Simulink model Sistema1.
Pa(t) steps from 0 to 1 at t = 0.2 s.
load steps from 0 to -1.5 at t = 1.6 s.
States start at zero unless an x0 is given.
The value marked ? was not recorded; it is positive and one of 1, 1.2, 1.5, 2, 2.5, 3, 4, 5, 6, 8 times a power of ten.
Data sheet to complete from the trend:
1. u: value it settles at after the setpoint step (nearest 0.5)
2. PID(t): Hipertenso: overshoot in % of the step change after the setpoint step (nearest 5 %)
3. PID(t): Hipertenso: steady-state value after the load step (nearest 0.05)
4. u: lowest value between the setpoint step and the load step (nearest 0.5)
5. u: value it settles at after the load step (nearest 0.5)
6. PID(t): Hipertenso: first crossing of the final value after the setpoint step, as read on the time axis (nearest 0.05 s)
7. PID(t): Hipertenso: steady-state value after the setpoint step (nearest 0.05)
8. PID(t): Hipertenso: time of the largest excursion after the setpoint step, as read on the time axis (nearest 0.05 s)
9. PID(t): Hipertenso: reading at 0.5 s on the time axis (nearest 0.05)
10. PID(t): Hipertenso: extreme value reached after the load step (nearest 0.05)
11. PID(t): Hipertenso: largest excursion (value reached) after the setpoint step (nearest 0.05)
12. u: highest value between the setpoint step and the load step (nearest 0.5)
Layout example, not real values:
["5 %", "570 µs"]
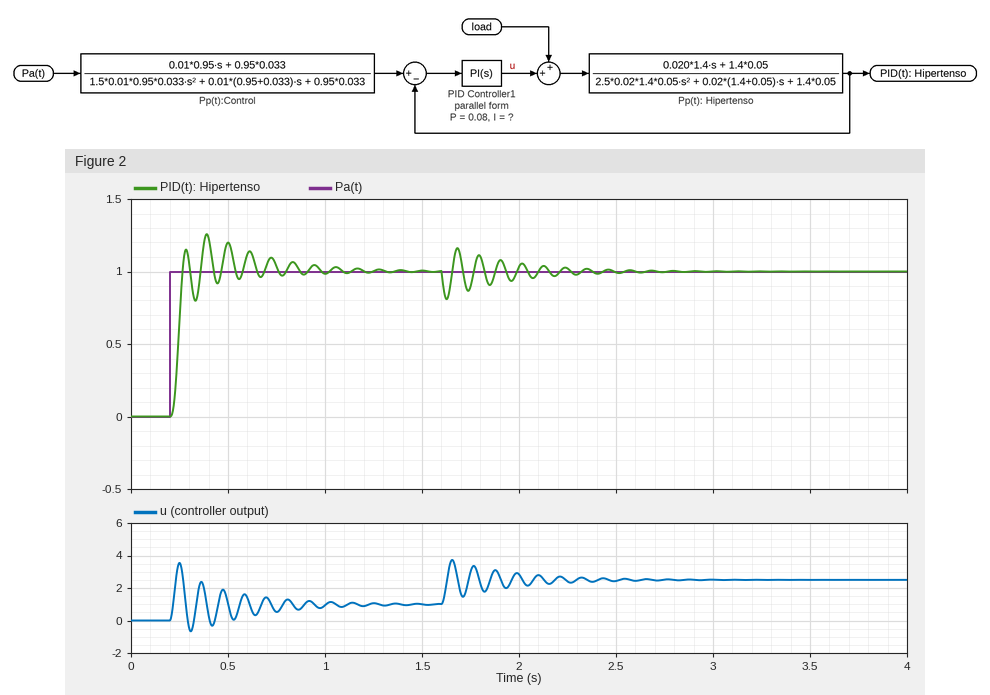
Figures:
["1.0", "25 %", "1.00", "-0.5", "2.5", "0.25 s", "1.00", "0.40 s", "1.20", "0.80", "1.25", "3.5"]
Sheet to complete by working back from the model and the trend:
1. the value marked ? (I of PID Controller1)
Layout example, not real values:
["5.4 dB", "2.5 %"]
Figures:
["400"]
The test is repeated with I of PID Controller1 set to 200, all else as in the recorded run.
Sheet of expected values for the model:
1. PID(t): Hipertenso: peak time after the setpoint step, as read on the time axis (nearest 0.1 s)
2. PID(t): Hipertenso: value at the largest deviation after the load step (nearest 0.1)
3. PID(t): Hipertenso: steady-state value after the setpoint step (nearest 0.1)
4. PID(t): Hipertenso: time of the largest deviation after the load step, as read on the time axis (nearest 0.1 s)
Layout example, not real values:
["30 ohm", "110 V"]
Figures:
["0.3 s", "0.7", "1.0", "1.6 s"]
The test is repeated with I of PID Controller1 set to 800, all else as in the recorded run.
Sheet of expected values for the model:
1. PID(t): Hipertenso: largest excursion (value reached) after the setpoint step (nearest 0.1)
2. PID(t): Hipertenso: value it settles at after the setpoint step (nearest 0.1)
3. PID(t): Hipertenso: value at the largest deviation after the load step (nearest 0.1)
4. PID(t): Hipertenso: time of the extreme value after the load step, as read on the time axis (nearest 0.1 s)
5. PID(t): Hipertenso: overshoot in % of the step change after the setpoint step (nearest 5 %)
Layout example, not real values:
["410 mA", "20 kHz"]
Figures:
["1.2", "1.0", "0.9", "1.6 s", "20 %"]
